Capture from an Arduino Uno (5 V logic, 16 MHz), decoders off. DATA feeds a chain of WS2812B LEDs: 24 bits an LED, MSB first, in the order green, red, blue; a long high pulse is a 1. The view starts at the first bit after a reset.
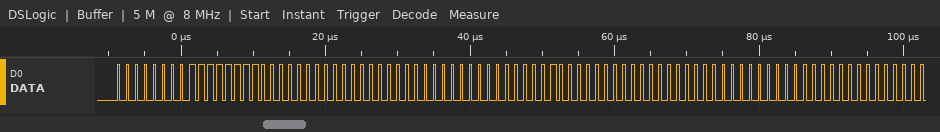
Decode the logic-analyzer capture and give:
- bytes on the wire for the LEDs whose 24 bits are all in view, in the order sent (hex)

00 FF 00 00 00 00 80 00 00
